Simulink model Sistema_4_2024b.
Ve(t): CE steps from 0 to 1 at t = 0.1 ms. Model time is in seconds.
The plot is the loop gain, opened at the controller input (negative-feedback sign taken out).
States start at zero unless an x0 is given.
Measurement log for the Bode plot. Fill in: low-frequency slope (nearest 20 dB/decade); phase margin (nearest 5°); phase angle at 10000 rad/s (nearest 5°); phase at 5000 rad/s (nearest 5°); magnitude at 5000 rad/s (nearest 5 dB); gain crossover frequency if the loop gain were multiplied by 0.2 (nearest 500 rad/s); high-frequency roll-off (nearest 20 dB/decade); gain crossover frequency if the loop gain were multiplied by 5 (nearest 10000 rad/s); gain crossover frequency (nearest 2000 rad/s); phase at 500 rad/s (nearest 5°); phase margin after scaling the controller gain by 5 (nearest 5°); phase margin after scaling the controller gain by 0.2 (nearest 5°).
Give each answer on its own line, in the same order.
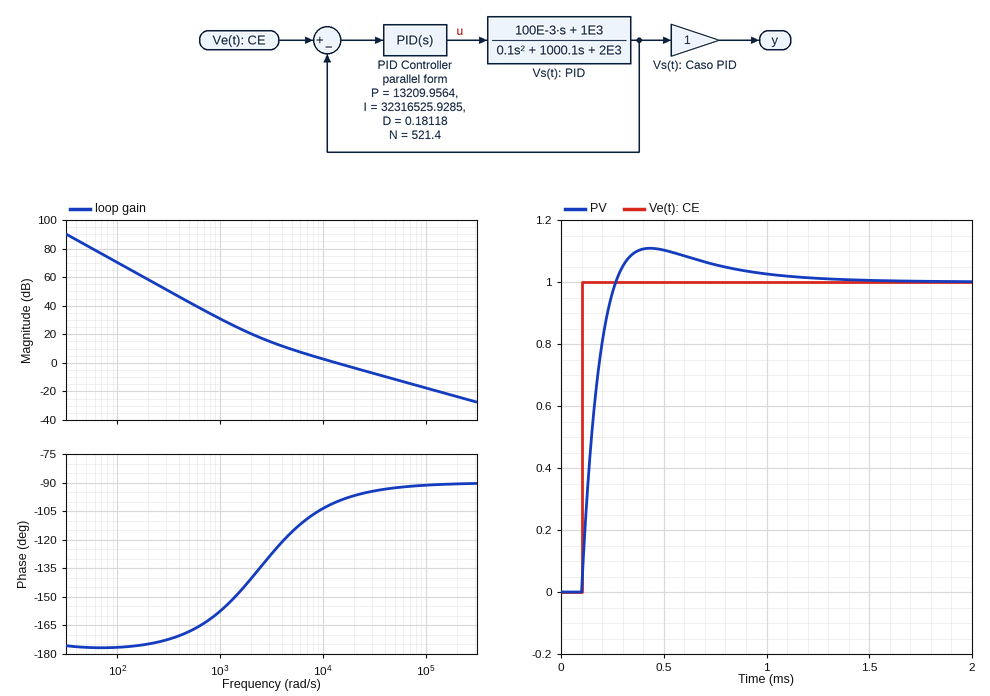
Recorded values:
-40 dB/decade
80°
-105°
-115°
10 dB
3500 rad/s
-20 dB/decade
70000 rad/s
14000 rad/s
-170°
90°
55°
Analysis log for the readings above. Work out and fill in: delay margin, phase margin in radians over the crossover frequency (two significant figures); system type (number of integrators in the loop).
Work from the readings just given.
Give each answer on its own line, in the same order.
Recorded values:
0.000100 s
2
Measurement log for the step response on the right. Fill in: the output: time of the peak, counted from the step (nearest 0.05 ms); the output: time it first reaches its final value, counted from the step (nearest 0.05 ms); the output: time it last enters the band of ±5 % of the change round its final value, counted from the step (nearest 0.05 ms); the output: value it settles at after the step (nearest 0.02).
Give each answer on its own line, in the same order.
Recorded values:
0.35 ms
0.15 ms
0.70 ms
1.00
